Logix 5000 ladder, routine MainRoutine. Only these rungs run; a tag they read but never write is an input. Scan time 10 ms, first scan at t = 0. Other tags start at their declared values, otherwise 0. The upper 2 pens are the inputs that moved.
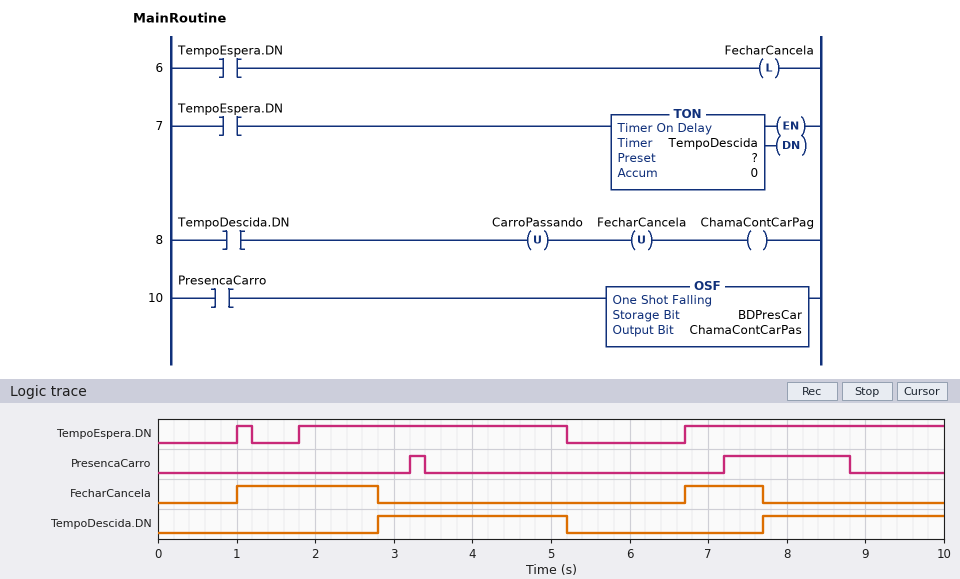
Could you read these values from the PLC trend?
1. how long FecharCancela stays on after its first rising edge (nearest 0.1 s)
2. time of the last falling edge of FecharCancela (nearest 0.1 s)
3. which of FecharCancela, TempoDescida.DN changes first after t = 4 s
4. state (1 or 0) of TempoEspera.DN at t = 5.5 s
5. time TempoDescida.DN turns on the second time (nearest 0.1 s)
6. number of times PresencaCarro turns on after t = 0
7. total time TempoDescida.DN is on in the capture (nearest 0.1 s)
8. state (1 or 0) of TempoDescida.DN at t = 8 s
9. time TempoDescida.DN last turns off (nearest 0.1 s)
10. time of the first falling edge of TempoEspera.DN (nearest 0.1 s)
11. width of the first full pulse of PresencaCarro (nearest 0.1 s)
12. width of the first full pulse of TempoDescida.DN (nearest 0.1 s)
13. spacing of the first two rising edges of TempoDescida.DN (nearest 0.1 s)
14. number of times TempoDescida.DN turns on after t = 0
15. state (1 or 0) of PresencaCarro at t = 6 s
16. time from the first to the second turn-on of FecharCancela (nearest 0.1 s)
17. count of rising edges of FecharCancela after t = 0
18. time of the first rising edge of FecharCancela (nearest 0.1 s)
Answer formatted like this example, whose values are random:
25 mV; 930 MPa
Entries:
1.8 s; 7.7 s; TempoDescida.DN; 0; 7.7 s; 2; 4.7 s; 1; 5.2 s; 1.2 s; 0.2 s; 2.4 s; 4.9 s; 2; 0; 5.7 s; 2; 1.0 s
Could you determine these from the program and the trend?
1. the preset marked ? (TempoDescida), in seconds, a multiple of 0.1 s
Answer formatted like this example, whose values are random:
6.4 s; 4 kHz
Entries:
1.0 s
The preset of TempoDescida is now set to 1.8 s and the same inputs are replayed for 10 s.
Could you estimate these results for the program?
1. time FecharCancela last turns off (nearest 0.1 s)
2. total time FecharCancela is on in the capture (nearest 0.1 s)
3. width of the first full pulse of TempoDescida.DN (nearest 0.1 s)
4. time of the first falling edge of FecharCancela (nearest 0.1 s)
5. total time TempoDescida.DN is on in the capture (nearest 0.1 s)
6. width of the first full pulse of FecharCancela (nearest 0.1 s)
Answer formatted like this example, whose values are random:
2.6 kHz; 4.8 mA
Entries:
8.5 s; 4.4 s; 1.6 s; 3.6 s; 3.1 s; 2.6 s
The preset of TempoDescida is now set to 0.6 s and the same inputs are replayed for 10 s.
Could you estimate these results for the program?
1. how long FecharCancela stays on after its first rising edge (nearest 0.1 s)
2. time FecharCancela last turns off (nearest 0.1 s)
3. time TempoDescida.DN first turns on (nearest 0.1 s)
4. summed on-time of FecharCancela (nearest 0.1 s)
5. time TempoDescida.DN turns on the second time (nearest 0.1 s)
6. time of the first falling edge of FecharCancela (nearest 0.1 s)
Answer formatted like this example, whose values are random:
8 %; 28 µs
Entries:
1.4 s; 7.3 s; 2.4 s; 2.0 s; 7.3 s; 2.4 s
